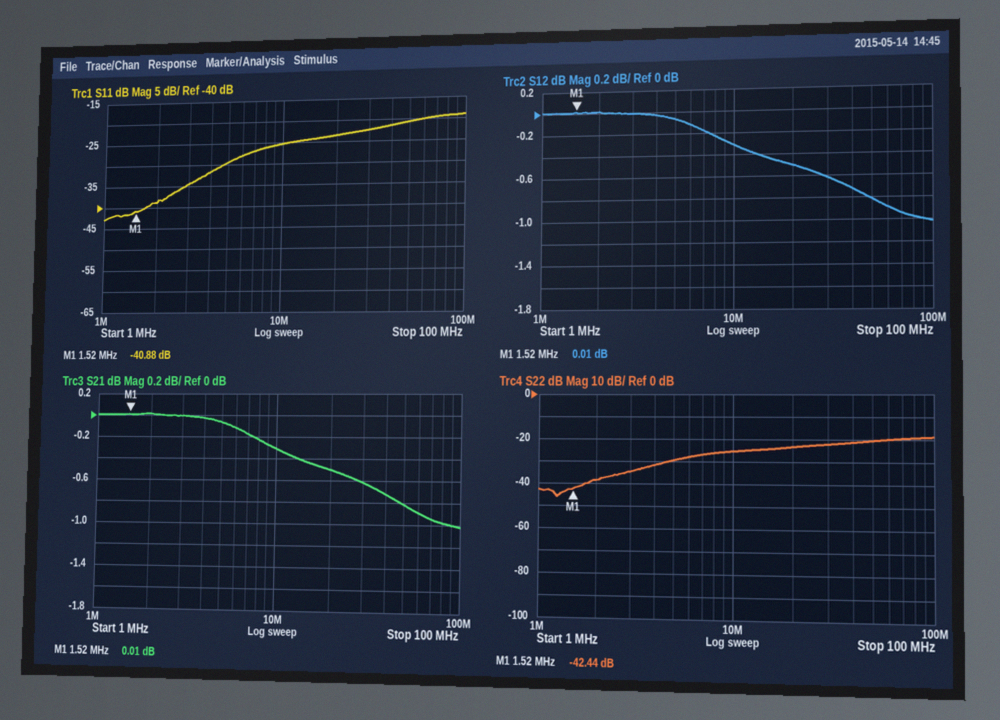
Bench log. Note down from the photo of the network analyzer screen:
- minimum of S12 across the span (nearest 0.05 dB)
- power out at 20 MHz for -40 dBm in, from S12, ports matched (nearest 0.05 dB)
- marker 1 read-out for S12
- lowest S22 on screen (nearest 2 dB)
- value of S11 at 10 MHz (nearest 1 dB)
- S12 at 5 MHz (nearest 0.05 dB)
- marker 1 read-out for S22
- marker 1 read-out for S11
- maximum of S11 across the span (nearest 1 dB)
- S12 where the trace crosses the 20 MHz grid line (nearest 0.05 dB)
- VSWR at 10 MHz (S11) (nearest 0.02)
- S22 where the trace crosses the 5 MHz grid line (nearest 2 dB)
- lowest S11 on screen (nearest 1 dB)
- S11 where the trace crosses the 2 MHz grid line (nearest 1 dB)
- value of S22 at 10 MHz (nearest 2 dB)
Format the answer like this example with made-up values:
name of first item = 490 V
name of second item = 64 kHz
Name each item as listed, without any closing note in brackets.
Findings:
minimum of S12 across the span = -1.00 dB
power out at 20 MHz for -40 dBm in, from S12, ports matched = -40.50 dBm
marker 1 read-out for S12 = 0.01 dB
lowest S22 on screen = -46 dB
value of S11 at 10 MHz = -25 dB
S12 at 5 MHz = -0.05 dB
marker 1 read-out for S22 = -42.44 dB
marker 1 read-out for S11 = -40.88 dB
maximum of S11 across the span = -19 dB
S12 where the trace crosses the 20 MHz grid line = -0.50 dB
VSWR at 10 MHz (S11) = 1.12
S22 where the trace crosses the 5 MHz grid line = -30 dB
lowest S11 on screen = -43 dB
S11 where the trace crosses the 2 MHz grid line = -39 dB
value of S22 at 10 MHz = -26 dB
